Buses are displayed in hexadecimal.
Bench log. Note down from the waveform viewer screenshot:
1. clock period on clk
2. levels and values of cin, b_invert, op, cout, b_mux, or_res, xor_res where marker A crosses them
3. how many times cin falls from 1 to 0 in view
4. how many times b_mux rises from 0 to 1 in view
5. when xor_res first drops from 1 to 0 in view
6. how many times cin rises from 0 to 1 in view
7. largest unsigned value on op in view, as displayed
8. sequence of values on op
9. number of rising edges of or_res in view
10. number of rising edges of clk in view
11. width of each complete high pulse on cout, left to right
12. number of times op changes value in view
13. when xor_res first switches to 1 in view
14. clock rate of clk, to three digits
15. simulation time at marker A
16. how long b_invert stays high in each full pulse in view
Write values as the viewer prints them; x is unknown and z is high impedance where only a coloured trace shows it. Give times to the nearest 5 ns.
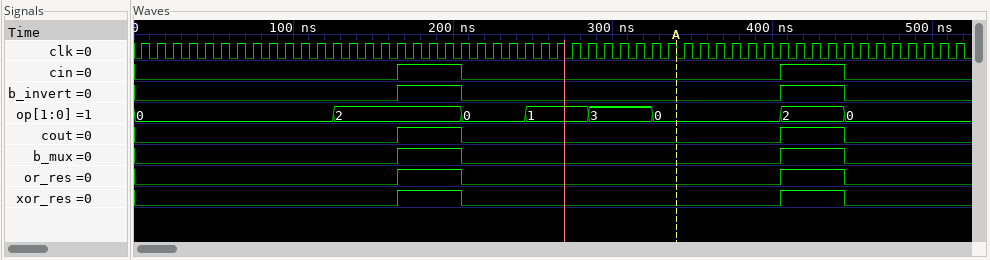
10 ns
cin=0, b_invert=0, op=0, cout=0, b_mux=0, or_res=0, xor_res=0
2
2
205 ns
2
3
0, 2, 0, 1, 3, 0, 2, 0
2
52
40 ns, 40 ns
7
165 ns
100 MHz
340 ns
40 ns, 40 ns
